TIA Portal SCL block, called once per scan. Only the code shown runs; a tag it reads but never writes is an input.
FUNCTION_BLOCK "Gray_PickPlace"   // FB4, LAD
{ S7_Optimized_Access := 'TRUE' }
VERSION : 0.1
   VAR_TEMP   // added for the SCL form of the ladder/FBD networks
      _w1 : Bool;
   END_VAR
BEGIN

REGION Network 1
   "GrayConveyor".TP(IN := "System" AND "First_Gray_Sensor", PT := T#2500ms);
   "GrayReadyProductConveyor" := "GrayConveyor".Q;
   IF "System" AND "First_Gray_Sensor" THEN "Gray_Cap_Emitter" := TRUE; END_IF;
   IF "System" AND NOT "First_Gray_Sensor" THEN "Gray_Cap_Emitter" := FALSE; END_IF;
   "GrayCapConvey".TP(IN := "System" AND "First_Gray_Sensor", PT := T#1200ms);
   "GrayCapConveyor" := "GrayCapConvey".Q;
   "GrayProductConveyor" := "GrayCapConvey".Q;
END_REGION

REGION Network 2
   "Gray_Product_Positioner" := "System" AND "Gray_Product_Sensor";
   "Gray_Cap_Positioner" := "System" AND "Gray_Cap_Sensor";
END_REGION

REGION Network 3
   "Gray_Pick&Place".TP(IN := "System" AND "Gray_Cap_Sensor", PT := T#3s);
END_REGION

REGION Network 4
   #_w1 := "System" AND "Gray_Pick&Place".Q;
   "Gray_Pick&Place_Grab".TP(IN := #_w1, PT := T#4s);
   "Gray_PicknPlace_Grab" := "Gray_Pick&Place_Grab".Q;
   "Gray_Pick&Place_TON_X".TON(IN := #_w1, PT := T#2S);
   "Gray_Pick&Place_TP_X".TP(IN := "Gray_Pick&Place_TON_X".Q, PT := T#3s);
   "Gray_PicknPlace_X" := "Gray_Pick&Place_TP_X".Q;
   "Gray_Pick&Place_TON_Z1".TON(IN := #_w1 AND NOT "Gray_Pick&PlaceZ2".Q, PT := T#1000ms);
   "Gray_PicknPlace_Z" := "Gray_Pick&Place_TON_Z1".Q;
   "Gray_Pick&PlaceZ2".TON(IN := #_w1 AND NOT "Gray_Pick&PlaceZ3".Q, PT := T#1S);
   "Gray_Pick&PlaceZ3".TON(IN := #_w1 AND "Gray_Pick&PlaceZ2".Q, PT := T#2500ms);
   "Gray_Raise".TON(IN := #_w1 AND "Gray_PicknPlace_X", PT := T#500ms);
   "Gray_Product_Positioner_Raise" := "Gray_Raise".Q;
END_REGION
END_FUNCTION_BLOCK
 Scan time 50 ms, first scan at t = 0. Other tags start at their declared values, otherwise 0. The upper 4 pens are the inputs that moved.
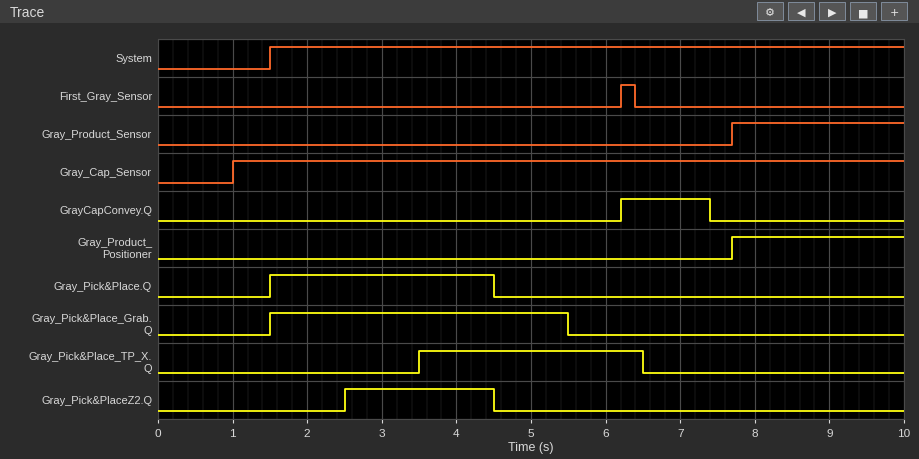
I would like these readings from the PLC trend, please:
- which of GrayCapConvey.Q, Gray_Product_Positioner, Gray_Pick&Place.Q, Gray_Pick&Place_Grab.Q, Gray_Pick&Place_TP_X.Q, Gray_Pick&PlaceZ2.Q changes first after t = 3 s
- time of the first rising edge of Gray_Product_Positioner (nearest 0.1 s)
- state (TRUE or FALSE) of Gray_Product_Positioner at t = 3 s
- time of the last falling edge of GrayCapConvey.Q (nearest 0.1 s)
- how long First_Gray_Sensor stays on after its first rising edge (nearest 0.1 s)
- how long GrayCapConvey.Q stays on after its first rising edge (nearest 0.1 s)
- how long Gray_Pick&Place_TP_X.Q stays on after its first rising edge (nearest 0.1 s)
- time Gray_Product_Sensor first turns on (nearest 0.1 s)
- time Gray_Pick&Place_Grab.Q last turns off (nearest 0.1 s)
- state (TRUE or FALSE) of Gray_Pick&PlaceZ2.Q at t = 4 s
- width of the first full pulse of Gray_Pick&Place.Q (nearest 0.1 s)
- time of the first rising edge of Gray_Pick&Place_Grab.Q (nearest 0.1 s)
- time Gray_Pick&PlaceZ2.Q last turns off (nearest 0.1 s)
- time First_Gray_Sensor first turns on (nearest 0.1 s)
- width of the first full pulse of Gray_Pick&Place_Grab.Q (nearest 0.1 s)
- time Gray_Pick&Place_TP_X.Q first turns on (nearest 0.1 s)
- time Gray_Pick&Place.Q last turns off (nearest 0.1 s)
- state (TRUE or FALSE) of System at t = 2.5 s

Gray_Pick&Place_TP_X.Q
7.7 s
FALSE
7.4 s
0.2 s
1.2 s
3.0 s
7.7 s
5.5 s
TRUE
3.0 s
1.5 s
4.5 s
6.2 s
4.0 s
3.5 s
4.5 s
TRUE
